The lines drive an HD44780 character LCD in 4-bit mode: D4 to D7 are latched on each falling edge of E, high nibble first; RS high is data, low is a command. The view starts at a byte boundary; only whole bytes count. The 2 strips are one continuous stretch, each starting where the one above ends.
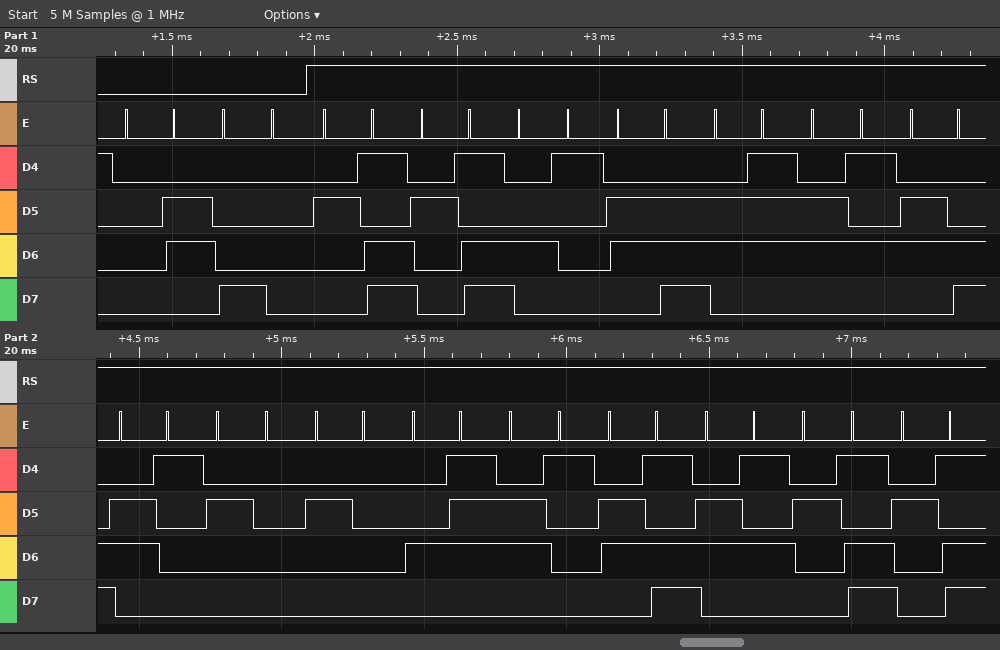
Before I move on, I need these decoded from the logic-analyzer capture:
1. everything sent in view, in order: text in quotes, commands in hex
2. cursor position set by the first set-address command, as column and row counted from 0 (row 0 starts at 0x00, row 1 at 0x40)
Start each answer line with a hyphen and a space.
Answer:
- 0x06 0x80 "--Angela  Game--"
- column 0, row 0
